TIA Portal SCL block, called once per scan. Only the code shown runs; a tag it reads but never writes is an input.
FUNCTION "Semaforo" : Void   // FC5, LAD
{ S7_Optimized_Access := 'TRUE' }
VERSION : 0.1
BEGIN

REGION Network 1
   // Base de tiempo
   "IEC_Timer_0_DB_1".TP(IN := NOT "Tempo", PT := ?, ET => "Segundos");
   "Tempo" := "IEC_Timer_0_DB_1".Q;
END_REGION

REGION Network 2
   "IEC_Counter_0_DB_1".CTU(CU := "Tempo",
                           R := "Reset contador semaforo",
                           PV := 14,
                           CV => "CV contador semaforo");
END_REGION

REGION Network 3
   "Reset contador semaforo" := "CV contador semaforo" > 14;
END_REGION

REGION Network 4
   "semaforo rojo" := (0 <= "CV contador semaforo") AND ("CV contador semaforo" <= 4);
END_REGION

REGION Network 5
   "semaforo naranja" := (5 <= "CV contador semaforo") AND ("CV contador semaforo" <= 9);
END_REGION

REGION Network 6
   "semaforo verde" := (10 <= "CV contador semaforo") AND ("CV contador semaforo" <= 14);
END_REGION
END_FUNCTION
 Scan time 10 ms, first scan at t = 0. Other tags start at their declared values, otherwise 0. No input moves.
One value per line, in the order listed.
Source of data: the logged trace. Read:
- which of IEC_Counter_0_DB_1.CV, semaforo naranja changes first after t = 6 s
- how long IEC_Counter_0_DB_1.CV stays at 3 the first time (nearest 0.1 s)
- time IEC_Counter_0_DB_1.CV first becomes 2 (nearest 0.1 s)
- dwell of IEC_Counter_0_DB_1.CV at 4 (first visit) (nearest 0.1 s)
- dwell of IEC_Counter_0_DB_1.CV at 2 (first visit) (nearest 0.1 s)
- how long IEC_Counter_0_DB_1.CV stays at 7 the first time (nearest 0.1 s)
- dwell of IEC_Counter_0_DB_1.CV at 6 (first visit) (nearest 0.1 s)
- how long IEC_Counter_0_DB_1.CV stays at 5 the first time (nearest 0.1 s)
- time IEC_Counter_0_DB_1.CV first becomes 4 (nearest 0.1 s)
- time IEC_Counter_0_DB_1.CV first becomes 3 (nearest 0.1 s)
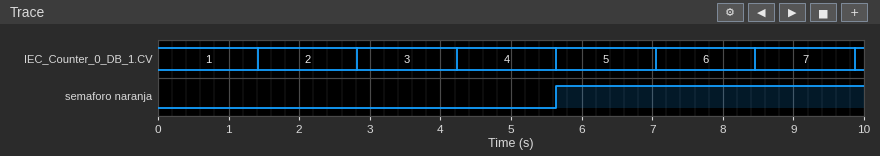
IEC_Counter_0_DB_1.CV
1.4 s
1.4 s
1.4 s
1.4 s
1.4 s
1.4 s
1.4 s
4.2 s
2.8 s
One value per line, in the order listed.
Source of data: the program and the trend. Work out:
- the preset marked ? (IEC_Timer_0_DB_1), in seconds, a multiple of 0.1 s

1.4 s
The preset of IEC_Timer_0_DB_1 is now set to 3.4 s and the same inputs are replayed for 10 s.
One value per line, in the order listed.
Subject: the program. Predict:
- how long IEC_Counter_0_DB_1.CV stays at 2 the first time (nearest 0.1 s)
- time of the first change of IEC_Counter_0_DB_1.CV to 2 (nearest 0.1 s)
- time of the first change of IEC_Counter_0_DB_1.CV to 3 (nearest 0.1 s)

3.4 s
3.4 s
6.8 s
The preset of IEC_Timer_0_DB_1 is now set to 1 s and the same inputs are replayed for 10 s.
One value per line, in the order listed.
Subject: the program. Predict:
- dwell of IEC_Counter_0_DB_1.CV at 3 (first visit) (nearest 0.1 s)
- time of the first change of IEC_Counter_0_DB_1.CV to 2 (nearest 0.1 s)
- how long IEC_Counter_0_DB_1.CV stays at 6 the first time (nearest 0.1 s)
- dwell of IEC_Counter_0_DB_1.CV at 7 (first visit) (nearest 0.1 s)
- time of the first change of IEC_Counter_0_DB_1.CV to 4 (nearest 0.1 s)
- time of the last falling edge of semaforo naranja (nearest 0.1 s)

1.0 s
1.0 s
1.0 s
1.0 s
3.0 s
9.1 s
